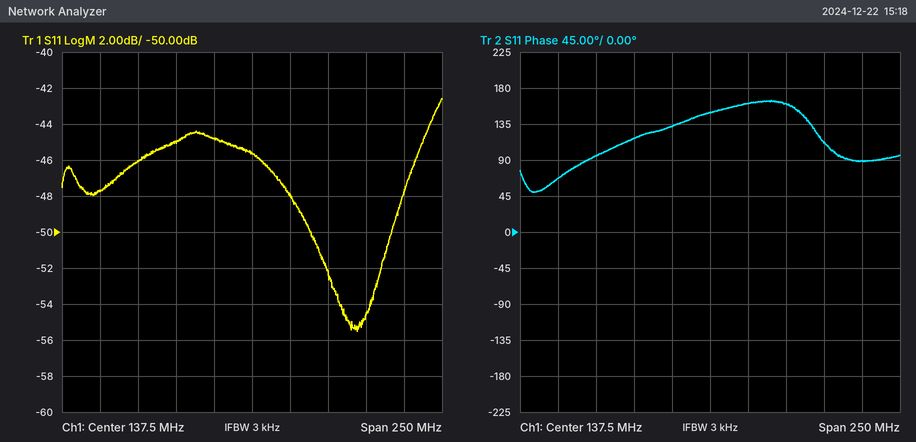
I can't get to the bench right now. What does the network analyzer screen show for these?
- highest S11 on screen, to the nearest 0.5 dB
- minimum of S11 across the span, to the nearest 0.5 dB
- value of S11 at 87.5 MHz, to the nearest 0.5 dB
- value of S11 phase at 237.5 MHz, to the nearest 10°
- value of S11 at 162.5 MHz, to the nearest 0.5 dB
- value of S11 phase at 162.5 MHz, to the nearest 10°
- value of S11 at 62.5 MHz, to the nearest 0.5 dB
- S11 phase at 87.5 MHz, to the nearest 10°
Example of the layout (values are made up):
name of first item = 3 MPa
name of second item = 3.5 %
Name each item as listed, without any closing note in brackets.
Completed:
highest S11 on screen, to the nearest 0.5 dB = -42.5 dB
minimum of S11 across the span, to the nearest 0.5 dB = -55.5 dB
value of S11 at 87.5 MHz, to the nearest 0.5 dB = -45.0 dB
value of S11 phase at 237.5 MHz, to the nearest 10° = 90°
value of S11 at 162.5 MHz, to the nearest 0.5 dB = -48.0 dB
value of S11 phase at 162.5 MHz, to the nearest 10° = 160°
value of S11 at 62.5 MHz, to the nearest 0.5 dB = -46.0 dB
S11 phase at 87.5 MHz, to the nearest 10° = 120°
